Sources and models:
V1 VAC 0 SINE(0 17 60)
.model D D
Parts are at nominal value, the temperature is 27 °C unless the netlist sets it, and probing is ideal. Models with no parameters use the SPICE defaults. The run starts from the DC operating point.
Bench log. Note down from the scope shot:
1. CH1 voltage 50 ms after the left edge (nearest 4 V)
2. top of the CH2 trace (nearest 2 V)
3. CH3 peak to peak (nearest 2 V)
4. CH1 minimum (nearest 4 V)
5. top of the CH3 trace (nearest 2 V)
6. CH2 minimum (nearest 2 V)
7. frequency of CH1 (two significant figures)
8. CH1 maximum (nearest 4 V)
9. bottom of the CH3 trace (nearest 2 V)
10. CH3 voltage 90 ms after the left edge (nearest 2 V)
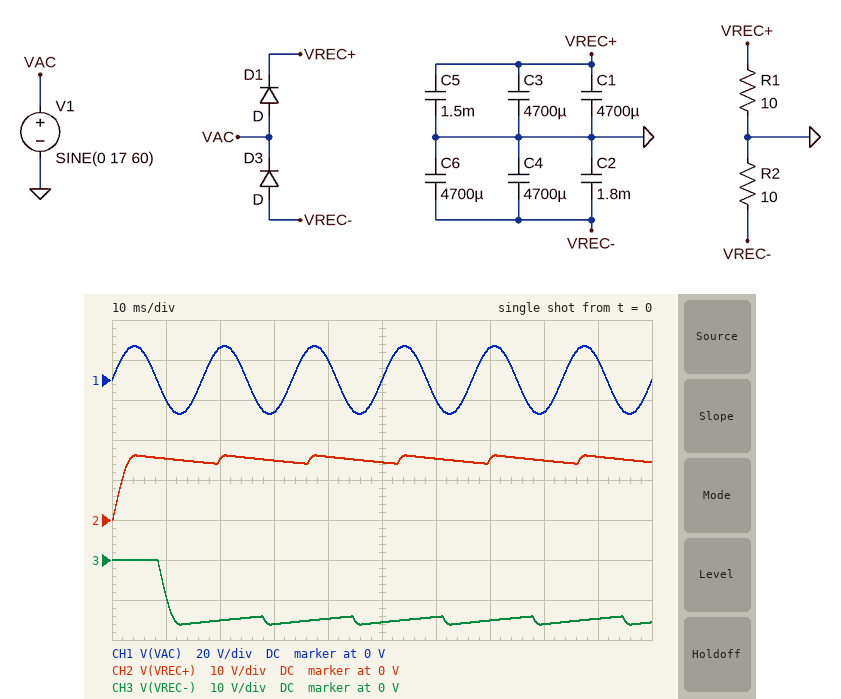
0 V
16 V
16 V
-16 V
0 V
0 V
60 Hz
16 V
-16 V
-14 V
